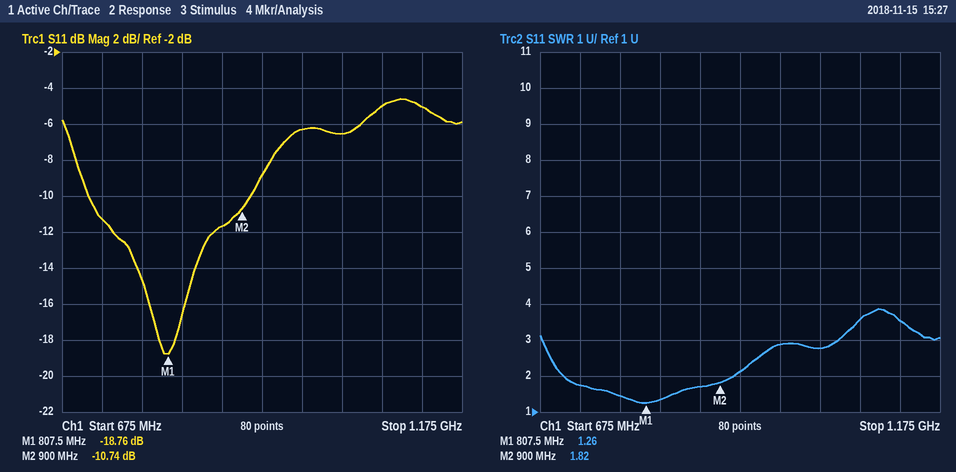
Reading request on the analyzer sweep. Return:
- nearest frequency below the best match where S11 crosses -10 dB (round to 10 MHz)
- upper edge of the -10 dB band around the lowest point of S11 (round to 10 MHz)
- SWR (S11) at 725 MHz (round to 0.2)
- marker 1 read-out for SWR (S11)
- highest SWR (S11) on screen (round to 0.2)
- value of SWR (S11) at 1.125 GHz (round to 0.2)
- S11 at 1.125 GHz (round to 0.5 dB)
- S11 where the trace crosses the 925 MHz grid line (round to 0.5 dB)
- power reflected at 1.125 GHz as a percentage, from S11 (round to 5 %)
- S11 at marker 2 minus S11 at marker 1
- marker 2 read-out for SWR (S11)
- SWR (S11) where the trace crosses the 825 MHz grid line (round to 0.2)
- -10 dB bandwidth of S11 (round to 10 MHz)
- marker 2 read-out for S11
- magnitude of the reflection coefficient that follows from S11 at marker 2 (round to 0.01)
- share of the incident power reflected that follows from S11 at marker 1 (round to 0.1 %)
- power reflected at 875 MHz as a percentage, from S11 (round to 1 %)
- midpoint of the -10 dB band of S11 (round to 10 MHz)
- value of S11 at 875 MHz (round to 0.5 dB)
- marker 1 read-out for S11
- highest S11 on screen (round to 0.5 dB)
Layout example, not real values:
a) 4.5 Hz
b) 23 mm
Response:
a) 710 MHz
b) 910 MHz
c) 1.8
d) 1.26
e) 3.8
f) 3.6
g) -5.0 dB
h) -9.0 dB
i) 30 %
j) 8.02 dB
k) 1.82
l) 1.4
m) 200 MHz
n) -10.74 dB
o) 0.29
p) 1.3 %
q) 7 %
r) 810 MHz
s) -11.5 dB
t) -18.76 dB
u) -4.5 dB
